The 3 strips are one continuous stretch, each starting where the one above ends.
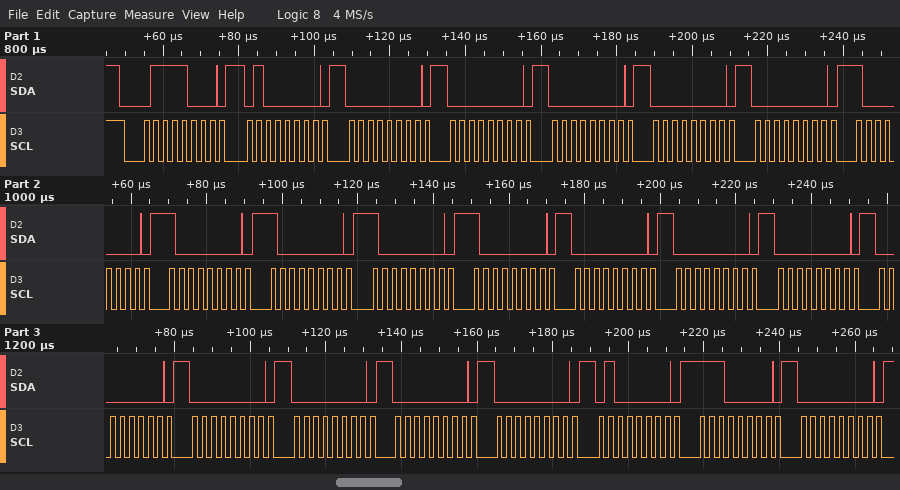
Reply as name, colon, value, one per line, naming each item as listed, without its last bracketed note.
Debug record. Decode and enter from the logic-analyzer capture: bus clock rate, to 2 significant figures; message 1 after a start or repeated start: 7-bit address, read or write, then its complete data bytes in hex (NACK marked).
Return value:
bus clock rate, to 2 significant figures: 400 kHz
message 1 after a start or repeated start: 7-bit address, read or write, then its complete data bytes in hex: 0x3C write: 40 00 00 00 00 00 80 80 80 80 80 00 00 00 00 00 00 00 00 40 E0 00
